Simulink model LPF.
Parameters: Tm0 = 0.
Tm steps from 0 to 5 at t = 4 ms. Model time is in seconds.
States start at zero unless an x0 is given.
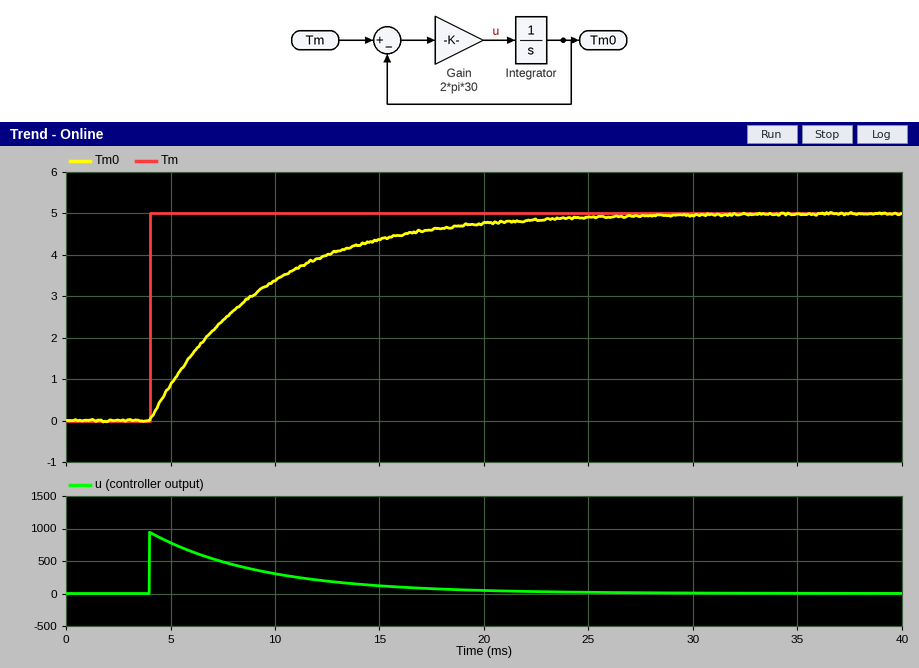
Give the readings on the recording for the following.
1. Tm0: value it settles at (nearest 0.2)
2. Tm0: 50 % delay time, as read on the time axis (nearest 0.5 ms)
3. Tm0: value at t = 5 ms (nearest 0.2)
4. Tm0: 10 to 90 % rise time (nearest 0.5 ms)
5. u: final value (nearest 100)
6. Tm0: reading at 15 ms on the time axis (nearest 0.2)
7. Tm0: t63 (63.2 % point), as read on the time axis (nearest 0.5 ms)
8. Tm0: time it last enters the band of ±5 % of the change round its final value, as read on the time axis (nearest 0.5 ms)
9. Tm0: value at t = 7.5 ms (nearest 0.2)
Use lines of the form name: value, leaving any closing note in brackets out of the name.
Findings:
Tm0: value it settles at: 5.0
Tm0: 50 % delay time, as read on the time axis: 7.5 ms
Tm0: value at t = 5 ms: 0.8
Tm0: 10 to 90 % rise time: 11.5 ms
u: final value: 0
Tm0: reading at 15 ms on the time axis: 4.4
Tm0: t63 (63.2 % point), as read on the time axis: 9.5 ms
Tm0: time it last enters the band of ±5 % of the change round its final value, as read on the time axis: 20.0 ms
Tm0: value at t = 7.5 ms: 2.4
